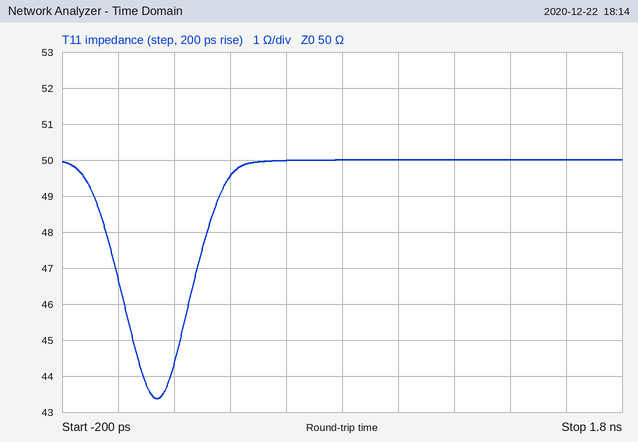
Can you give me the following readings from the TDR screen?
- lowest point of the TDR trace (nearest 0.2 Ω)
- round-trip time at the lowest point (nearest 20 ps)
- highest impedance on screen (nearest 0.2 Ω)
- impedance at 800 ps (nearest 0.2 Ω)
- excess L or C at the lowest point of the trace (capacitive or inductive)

43.4 Ω
140 ps
50.0 Ω
50.0 Ω
capacitive
